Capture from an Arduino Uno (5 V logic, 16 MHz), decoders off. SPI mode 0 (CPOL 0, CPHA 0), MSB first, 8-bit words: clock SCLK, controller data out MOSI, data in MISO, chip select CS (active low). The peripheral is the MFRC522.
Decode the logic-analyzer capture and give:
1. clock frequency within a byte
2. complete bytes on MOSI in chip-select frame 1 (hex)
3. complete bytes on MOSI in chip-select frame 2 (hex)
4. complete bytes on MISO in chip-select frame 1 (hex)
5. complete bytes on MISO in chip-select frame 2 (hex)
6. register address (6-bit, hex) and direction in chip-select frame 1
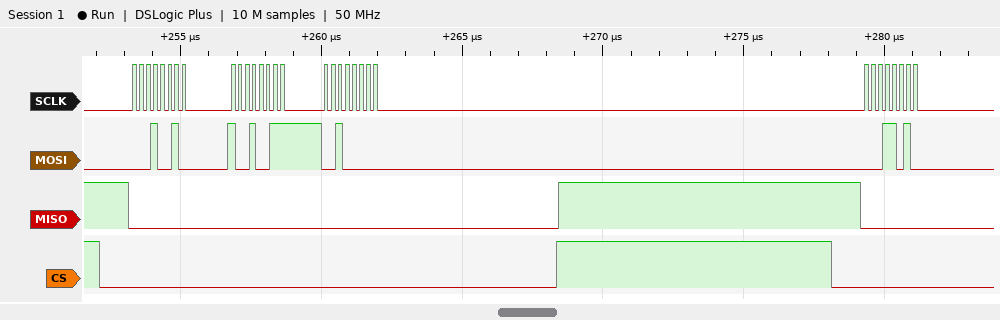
4 MHz
12 93 20
1A
00 00 00
00
0x09 write
